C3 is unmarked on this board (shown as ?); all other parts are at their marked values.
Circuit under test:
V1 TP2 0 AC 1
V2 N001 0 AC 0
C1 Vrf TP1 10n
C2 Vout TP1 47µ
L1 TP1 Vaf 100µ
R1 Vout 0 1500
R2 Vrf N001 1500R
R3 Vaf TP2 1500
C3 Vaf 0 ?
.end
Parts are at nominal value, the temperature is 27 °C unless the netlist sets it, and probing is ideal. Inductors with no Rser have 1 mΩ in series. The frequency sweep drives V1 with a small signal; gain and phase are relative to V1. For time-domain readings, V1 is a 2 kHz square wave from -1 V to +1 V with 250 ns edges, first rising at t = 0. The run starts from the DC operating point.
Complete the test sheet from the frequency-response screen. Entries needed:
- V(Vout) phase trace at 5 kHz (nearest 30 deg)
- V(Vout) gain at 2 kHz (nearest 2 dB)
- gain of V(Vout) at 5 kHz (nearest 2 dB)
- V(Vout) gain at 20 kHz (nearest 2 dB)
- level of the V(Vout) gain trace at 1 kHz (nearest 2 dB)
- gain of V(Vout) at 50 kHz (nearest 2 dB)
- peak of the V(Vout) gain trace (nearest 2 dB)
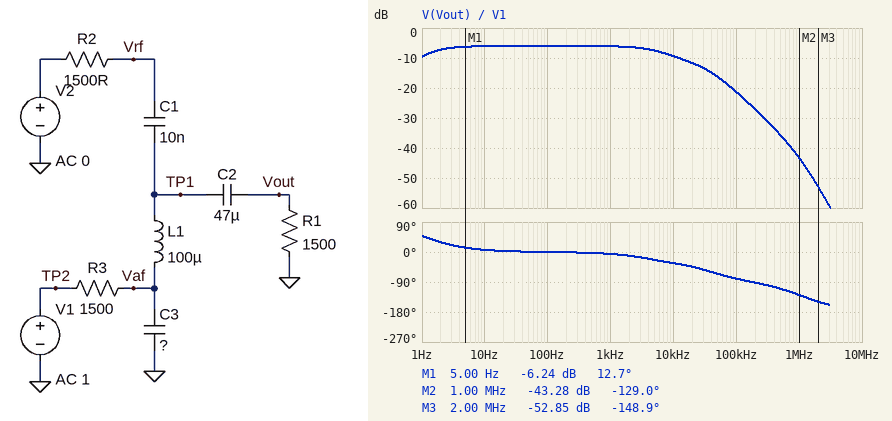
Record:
-30 deg
-6 dB
-8 dB
-12 dB
-6 dB
-16 dB
-6 dB
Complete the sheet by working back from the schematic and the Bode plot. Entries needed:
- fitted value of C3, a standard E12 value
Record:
12 nF
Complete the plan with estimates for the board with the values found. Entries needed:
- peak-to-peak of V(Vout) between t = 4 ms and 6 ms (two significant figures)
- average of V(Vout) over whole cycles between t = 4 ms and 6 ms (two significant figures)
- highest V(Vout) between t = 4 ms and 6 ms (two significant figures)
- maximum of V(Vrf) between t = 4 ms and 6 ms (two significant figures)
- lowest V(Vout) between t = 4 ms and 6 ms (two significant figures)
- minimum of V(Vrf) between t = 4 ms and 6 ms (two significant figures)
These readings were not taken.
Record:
1.0 V
480 mV
980 mV
390 mV
-21 mV
-390 mV
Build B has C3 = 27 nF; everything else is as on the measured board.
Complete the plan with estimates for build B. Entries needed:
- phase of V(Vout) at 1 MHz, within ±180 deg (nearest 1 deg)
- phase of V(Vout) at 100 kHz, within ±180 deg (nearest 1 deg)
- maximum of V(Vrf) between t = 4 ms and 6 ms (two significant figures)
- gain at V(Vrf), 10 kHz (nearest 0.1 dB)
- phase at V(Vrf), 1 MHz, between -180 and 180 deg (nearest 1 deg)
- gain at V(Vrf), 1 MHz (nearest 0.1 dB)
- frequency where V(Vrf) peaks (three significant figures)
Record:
-130 deg
-88 deg
280 mV
-15.1 dB
-129 deg
-50.4 dB
9.18 kHz
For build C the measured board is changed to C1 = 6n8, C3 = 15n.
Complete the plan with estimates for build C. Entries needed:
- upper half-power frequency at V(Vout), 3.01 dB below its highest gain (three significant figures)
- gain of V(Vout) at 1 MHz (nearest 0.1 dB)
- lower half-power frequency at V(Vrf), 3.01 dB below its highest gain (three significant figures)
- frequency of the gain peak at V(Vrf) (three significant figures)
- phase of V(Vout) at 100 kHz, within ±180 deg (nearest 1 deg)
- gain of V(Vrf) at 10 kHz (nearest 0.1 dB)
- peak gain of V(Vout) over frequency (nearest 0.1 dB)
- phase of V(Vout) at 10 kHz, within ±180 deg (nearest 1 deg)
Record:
9.08 kHz
-45.2 dB
5.27 kHz
15.0 kHz
-83 deg
-14.8 dB
-6.0 dB
-39 deg
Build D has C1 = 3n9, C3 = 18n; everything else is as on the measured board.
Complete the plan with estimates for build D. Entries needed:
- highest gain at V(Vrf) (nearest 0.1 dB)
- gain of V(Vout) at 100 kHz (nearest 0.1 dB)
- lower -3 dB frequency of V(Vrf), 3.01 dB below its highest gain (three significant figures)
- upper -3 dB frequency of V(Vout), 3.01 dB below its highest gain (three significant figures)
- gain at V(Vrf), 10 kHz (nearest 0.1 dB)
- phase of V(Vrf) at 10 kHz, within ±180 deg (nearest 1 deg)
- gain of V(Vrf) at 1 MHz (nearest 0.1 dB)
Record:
-17.6 dB
-24.7 dB
6.31 kHz
9.36 kHz
-18.6 dB
26 deg
-46.8 dB
